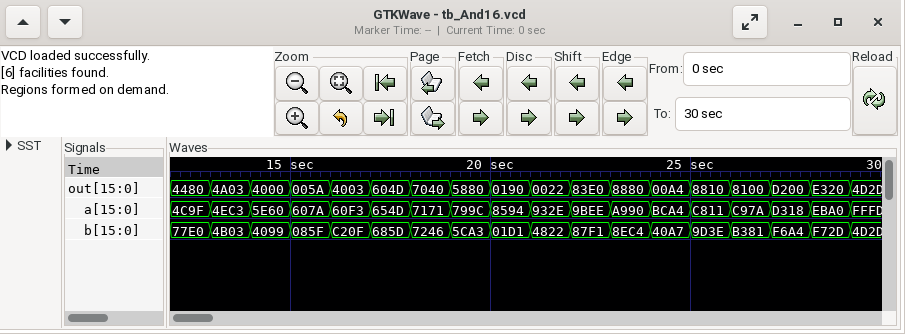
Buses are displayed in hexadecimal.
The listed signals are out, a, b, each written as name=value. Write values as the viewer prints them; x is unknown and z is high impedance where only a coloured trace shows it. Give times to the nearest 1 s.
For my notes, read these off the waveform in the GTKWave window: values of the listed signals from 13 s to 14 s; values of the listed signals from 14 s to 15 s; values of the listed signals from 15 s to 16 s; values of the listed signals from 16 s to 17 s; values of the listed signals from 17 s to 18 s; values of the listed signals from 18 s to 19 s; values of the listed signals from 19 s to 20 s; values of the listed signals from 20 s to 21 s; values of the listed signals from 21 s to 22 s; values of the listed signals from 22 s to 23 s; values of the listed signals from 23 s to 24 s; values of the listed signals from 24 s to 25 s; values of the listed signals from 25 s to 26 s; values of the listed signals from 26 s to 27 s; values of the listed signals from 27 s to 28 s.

out=4A03, a=4EC3, b=4B03
out=4000, a=5E60, b=4099
out=005A, a=607A, b=085F
out=4003, a=60F3, b=C20F
out=604D, a=654D, b=685D
out=7040, a=7171, b=7246
out=5880, a=799C, b=5CA3
out=0190, a=8594, b=01D1
out=0022, a=932E, b=4822
out=83E0, a=9BEE, b=87F1
out=8880, a=A990, b=8EC4
out=00A4, a=BCA4, b=40A7
out=8810, a=C811, b=9D3E
out=8100, a=C97A, b=B381
out=D200, a=D318, b=F6A4
